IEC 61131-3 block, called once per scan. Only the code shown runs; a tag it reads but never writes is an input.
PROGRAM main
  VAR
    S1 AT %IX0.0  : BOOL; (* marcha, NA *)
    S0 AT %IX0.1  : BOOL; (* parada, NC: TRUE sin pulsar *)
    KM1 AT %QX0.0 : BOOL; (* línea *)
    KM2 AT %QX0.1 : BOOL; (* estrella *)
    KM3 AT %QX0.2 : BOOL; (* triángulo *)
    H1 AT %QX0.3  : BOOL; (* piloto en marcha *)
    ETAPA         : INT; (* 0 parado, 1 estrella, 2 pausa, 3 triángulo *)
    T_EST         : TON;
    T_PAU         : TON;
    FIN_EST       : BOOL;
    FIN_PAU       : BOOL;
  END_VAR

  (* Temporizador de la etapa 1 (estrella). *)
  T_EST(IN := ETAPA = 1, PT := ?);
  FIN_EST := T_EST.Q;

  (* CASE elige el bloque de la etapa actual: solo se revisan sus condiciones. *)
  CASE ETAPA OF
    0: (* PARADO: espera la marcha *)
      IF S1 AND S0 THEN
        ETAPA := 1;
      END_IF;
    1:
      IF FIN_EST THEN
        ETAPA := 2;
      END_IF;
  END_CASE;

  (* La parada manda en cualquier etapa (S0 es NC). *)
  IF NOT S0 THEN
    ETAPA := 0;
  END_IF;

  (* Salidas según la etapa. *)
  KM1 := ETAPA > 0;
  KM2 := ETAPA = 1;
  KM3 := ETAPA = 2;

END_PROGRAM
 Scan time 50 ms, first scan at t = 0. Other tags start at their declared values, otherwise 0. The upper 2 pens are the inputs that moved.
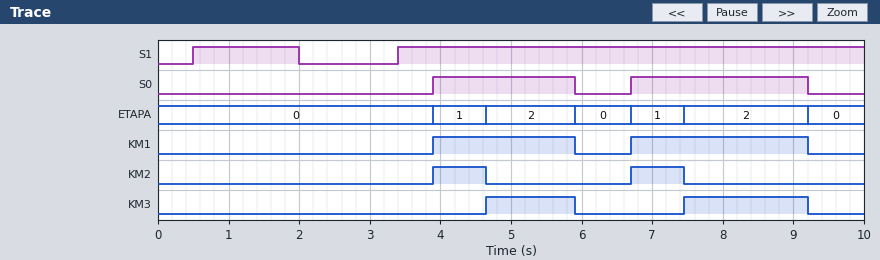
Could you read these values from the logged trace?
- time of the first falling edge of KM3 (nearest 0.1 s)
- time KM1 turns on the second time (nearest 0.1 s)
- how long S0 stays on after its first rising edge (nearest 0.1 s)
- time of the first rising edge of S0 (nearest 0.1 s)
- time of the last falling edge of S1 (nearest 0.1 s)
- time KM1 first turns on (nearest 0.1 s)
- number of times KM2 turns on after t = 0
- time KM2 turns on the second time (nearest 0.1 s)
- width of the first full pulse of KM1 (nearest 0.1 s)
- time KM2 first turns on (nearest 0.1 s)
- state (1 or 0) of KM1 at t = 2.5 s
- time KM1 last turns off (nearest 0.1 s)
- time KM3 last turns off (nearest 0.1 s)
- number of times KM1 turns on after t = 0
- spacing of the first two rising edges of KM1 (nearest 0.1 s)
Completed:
5.9 s
6.7 s
2.0 s
3.9 s
2.0 s
3.9 s
2
6.7 s
2.0 s
3.9 s
0
9.2 s
9.2 s
2
2.8 s
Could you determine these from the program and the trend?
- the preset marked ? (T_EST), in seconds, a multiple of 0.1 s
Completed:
0.7 s
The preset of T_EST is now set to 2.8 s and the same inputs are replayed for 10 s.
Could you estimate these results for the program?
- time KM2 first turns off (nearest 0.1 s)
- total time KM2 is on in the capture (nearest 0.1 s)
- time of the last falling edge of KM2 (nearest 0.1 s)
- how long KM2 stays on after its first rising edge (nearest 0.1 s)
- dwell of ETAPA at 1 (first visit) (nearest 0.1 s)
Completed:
5.9 s
4.5 s
9.2 s
2.0 s
2.0 s
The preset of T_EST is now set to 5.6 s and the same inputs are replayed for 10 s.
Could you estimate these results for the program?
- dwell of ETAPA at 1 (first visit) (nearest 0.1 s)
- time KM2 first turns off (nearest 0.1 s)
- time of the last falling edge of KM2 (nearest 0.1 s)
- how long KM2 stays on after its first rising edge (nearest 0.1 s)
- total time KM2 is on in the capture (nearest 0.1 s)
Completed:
2.0 s
5.9 s
9.2 s
2.0 s
4.5 s
